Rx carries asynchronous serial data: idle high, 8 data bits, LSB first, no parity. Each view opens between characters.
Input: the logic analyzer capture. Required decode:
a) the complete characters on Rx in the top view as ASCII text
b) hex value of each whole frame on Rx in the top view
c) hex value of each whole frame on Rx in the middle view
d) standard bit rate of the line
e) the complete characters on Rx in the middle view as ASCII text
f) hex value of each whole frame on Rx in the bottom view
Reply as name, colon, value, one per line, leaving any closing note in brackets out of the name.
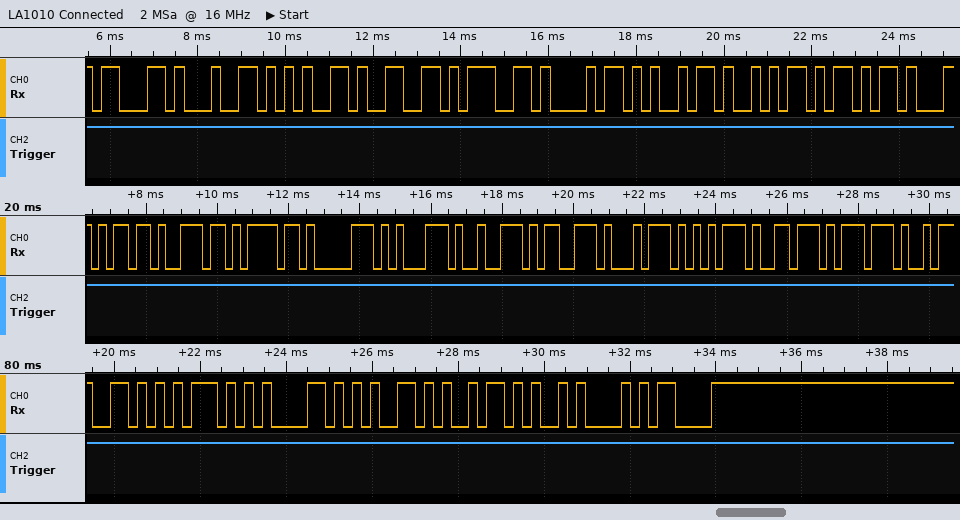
the complete characters on Rx in the top view as ASCII text: "cdefghijk"
hex value of each whole frame on Rx in the top view: 63, 64, 65, 66, 67, 68, 69, 6A, 6B
hex value of each whole frame on Rx in the middle view: 6D, 6E, 6F, 70, 71, 72, 73, 74, 75, 76, 77
standard bit rate of the line: 4800 baud
the complete characters on Rx in the middle view as ASCII text: "mnopqrstuvw"
hex value of each whole frame on Rx in the bottom view: 56, 57, 58, 59, 5A, 0A, 0D
